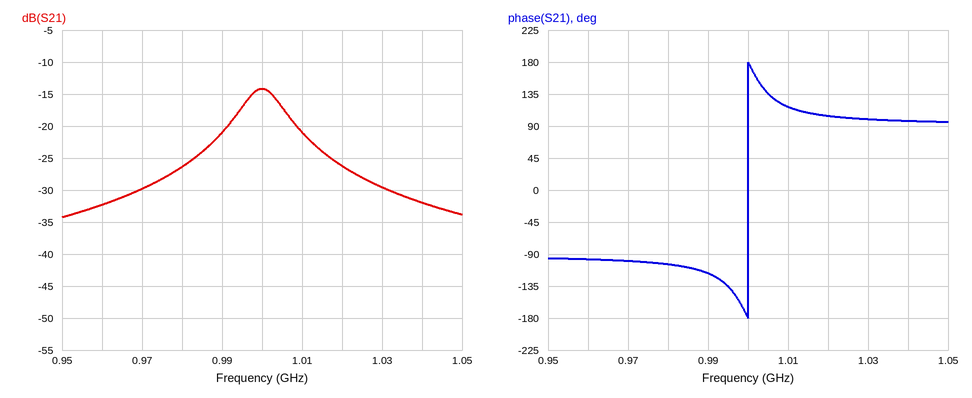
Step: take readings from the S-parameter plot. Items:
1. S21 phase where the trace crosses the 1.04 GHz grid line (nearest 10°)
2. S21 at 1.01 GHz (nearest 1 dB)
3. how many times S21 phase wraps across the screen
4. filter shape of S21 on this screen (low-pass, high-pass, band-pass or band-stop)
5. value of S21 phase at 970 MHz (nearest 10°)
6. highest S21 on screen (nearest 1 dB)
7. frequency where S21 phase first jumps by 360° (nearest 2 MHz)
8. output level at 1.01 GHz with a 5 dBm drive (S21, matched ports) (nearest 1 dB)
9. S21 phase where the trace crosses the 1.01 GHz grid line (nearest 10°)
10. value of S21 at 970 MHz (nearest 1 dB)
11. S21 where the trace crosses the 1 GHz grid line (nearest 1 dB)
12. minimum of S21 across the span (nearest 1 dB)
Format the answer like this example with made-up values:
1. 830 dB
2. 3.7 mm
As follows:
1. 100°
2. -21 dB
3. 1
4. band-pass
5. -100°
6. -14 dB
7. 1.000 GHz
8. -16 dBm
9. 120°
10. -30 dB
11. -14 dB
12. -34 dB
